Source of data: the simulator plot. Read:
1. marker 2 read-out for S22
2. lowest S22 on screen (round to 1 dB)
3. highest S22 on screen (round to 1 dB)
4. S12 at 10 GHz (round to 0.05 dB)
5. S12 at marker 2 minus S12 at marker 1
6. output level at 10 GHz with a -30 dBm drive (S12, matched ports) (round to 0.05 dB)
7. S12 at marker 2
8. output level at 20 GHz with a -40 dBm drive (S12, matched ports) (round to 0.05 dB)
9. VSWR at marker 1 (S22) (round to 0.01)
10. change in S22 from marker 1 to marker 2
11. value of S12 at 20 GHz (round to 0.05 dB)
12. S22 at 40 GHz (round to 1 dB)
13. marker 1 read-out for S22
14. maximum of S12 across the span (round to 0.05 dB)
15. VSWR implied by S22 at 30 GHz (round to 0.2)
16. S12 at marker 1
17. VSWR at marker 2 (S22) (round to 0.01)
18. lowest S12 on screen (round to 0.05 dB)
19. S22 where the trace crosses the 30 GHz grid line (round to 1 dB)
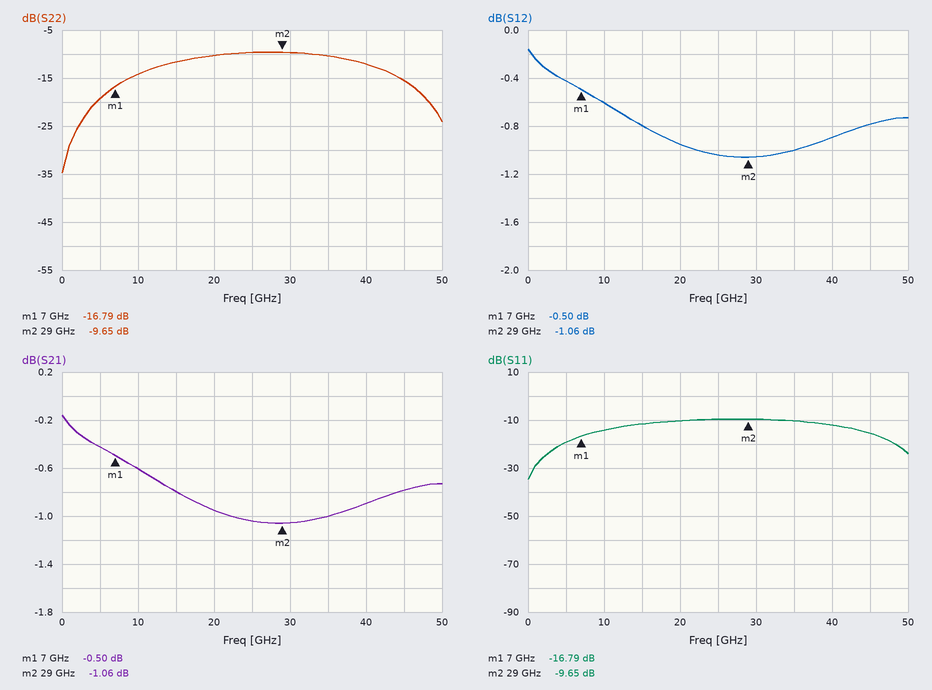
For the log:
-9.65 dB
-35 dB
-10 dB
-0.60 dB
-0.56 dB
-30.60 dBm
-1.06 dB
-40.95 dBm
1.34
7.14 dB
-0.95 dB
-12 dB
-16.79 dB
-0.15 dB
2.0
-0.50 dB
1.98
-1.05 dB
-10 dB
